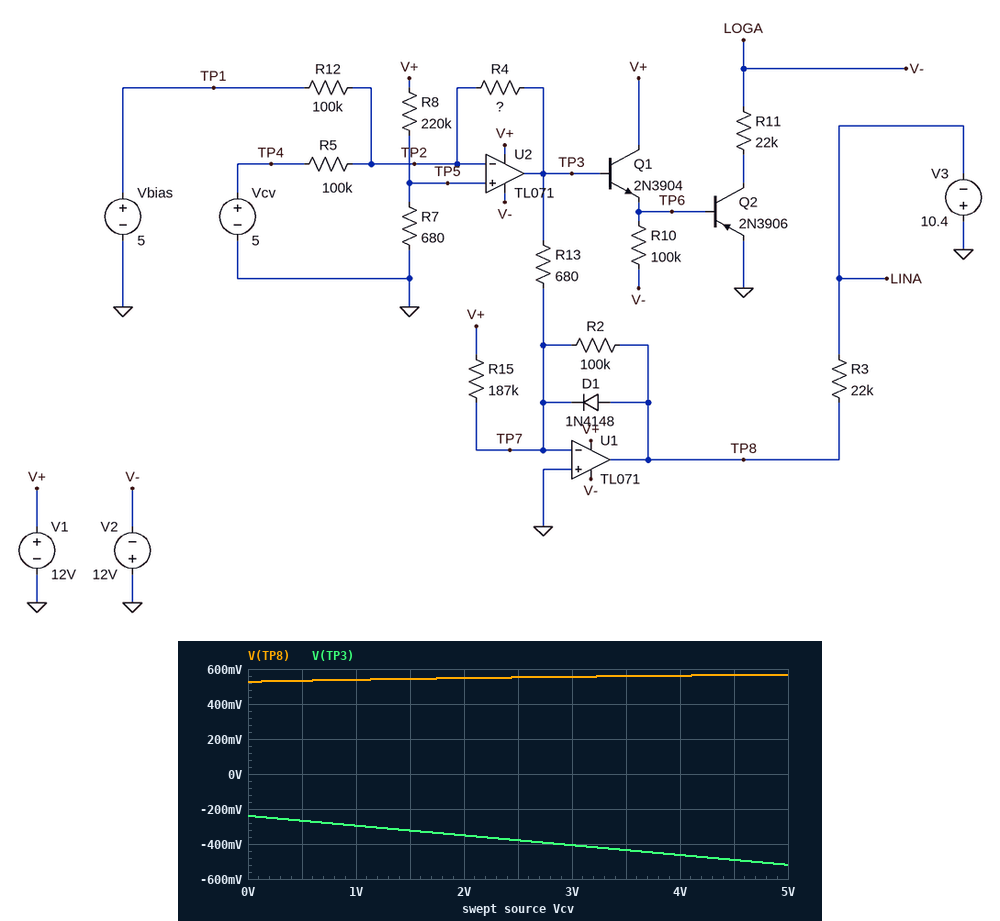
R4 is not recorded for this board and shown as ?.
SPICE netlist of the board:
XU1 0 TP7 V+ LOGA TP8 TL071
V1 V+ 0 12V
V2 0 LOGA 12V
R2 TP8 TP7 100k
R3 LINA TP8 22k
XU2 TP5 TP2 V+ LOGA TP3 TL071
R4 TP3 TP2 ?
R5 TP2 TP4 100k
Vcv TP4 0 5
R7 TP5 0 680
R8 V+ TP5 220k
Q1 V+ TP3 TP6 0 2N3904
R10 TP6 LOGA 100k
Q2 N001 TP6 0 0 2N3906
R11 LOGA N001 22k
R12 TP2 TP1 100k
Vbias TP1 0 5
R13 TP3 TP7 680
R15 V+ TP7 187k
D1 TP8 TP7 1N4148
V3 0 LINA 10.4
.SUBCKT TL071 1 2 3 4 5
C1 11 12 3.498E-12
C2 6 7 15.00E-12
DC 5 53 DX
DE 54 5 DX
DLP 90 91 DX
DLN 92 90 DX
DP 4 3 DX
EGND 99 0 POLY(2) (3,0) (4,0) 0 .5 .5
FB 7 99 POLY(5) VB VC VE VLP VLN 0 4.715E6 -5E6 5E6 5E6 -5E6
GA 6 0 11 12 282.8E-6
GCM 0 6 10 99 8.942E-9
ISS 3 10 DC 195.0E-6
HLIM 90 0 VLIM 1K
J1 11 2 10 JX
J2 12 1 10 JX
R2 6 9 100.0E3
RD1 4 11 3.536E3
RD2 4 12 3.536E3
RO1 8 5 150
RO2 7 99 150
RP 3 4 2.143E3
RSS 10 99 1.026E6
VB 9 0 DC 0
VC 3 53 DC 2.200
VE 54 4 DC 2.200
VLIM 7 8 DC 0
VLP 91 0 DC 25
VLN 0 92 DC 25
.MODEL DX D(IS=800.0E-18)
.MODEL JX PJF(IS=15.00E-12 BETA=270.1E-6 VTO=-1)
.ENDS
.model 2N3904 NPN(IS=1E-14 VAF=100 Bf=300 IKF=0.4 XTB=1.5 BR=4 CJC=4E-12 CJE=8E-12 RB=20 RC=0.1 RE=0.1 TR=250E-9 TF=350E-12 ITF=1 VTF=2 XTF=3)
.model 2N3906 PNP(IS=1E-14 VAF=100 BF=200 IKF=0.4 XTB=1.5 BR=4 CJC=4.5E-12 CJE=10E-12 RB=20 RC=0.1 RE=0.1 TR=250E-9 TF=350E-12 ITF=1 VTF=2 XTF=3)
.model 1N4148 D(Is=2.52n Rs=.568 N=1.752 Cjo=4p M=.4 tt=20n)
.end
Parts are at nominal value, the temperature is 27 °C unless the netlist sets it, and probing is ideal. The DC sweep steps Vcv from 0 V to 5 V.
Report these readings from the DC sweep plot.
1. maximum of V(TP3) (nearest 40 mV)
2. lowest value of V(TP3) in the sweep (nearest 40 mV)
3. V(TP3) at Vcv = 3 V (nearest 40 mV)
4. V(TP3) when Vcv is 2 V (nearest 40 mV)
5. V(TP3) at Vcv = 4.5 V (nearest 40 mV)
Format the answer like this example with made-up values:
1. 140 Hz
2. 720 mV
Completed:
1. -240 mV
2. -520 mV
3. -400 mV
4. -360 mV
5. -480 mV
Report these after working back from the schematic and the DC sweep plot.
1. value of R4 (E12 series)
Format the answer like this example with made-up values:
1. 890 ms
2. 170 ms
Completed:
1. 5.6 kΩ
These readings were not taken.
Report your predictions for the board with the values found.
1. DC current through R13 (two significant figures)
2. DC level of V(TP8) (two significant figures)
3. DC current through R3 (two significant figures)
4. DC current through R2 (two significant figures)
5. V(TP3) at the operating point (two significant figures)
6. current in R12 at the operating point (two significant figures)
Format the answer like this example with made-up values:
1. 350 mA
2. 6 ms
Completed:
1. 760 µA
2. 570 mV
3. 500 µA
4. 5.7 µA
5. -520 mV
6. 50 µA
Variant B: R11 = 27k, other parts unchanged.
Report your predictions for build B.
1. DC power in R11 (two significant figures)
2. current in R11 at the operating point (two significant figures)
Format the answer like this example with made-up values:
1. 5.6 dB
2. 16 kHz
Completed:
1. 5.3 mW
2. 440 µA
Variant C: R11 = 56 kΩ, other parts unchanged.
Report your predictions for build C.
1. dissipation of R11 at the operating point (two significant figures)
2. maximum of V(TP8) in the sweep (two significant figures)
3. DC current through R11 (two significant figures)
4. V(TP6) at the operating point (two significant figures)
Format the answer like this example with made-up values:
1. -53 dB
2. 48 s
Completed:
1. 2.6 mW
2. 570 mV
3. 210 µA
4. -650 mV
